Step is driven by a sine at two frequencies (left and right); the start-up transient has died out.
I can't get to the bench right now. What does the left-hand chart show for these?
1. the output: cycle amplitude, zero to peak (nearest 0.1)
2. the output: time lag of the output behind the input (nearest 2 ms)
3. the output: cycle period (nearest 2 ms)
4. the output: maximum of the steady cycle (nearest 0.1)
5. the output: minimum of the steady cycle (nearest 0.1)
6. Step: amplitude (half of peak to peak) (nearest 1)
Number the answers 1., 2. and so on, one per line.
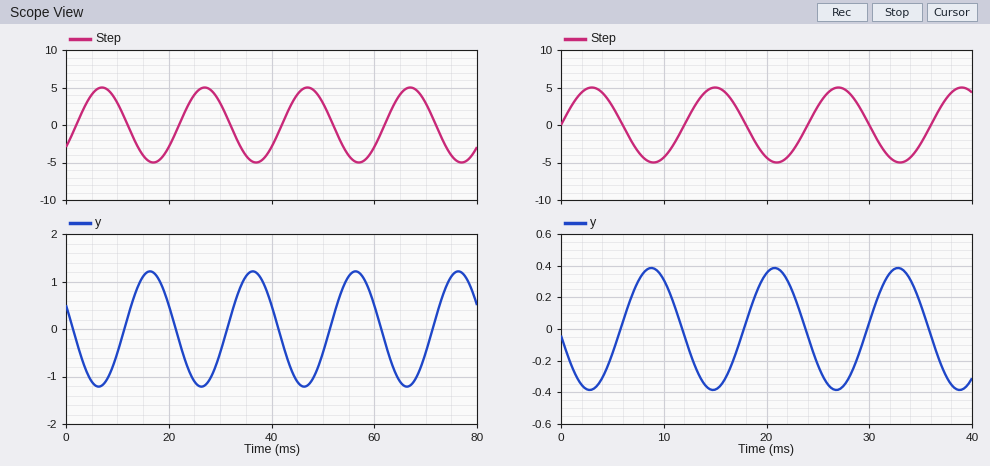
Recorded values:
1. 1.2
2. 10 ms
3. 20 ms
4. 1.2
5. -1.2
6. 5
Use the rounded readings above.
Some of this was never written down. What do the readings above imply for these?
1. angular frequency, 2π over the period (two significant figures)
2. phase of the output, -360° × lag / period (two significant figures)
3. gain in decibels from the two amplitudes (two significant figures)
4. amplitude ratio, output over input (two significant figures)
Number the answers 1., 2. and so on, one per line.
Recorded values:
1. 0.31 rad/ms
2. -180°
3. -12 dB
4. 0.24
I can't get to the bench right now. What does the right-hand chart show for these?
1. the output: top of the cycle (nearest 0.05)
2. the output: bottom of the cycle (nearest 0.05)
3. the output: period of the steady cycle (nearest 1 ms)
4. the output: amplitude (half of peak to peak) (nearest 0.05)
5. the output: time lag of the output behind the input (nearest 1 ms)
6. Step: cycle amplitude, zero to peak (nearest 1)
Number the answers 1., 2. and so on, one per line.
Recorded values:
1. 0.40
2. -0.40
3. 12 ms
4. 0.40
5. 6 ms
6. 5
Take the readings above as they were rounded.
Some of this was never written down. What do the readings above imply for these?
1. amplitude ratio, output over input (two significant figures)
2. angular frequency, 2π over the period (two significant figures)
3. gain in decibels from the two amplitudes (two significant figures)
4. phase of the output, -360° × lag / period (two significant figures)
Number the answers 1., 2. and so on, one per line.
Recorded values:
1. 0.080
2. 0.52 rad/ms
3. -22 dB
4. -180°
